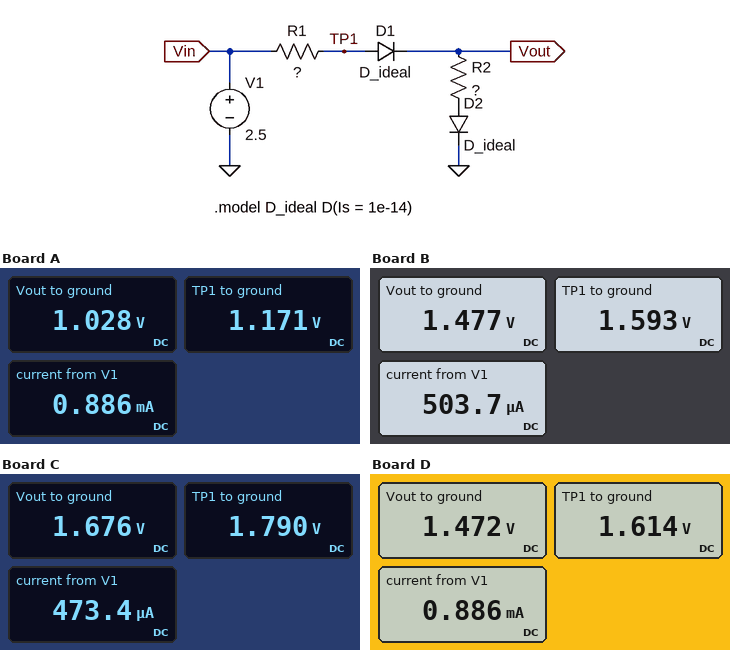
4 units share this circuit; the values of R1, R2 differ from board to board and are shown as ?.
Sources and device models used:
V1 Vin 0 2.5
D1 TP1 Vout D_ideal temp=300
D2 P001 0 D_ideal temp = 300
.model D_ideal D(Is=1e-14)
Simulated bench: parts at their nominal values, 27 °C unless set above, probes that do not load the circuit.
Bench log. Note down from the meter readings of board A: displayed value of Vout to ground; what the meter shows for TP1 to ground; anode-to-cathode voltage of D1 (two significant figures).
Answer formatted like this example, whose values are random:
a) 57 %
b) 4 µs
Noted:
a) 1.028 V
b) 1.171 V
c) 140 mV
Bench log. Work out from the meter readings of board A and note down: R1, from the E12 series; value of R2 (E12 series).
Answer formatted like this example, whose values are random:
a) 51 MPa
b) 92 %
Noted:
a) 1.5 kΩ
b) 1 kΩ
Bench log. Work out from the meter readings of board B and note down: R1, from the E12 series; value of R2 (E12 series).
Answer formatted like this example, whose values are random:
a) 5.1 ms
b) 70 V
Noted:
a) 1.8 kΩ
b) 2.7 kΩ
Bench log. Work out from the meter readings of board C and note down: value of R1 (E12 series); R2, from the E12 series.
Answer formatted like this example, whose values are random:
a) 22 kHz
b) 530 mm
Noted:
a) 1.5 kΩ
b) 3.3 kΩ
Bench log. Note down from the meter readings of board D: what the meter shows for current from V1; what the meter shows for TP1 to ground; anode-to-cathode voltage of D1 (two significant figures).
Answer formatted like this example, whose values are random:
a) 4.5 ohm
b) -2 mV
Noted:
a) 0.886 mA
b) 1.614 V
c) 140 mV
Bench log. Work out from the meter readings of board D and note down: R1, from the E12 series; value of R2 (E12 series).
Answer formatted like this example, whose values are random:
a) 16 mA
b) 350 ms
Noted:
a) 1 kΩ
b) 1.5 kΩ
